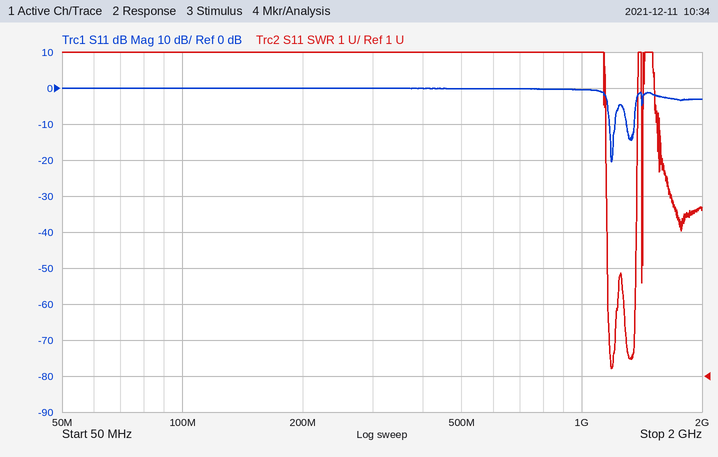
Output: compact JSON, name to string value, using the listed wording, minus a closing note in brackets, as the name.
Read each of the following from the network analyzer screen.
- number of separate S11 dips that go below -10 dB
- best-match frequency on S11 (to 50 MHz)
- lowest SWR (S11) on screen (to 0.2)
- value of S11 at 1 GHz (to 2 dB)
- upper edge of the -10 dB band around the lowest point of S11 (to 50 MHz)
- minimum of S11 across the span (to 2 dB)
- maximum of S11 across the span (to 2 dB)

{"number of separate S11 dips that go below -10 dB": "2", "best-match frequency on S11": "1.20 GHz", "lowest SWR (S11) on screen": "1.2", "value of S11 at 1 GHz": "0 dB", "upper edge of the -10 dB band around the lowest point of S11": "1.20 GHz", "minimum of S11 across the span": "-20 dB", "maximum of S11 across the span": "0 dB"}
